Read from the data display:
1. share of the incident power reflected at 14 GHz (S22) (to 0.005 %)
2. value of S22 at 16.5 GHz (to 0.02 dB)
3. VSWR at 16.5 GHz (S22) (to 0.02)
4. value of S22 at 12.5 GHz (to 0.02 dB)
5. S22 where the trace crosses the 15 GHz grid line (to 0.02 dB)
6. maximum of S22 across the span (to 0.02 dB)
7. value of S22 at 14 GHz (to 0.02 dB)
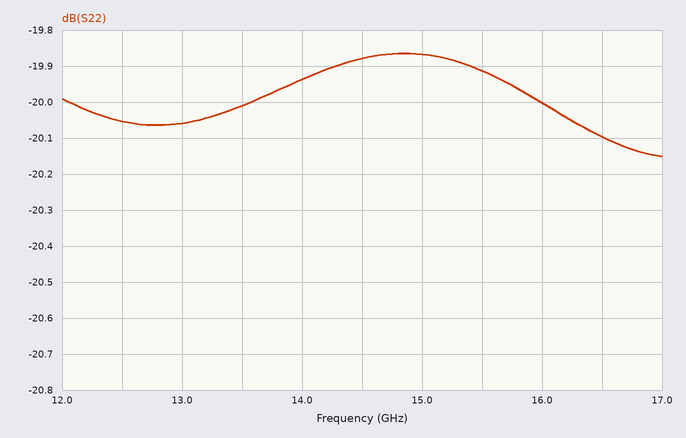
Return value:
1.015 %
-20.10 dB
1.22
-20.06 dB
-19.86 dB
-19.86 dB
-19.94 dB
